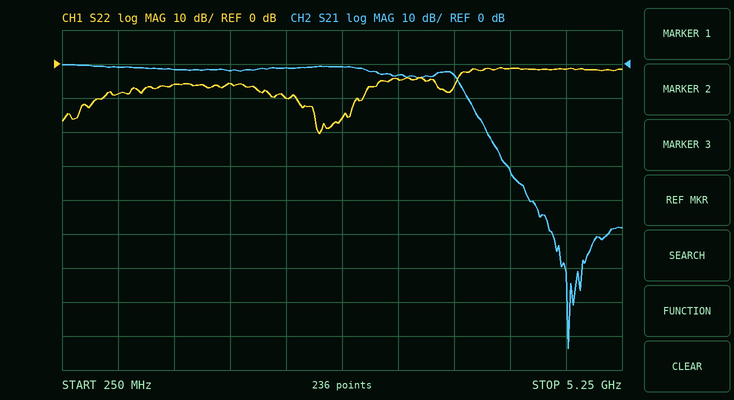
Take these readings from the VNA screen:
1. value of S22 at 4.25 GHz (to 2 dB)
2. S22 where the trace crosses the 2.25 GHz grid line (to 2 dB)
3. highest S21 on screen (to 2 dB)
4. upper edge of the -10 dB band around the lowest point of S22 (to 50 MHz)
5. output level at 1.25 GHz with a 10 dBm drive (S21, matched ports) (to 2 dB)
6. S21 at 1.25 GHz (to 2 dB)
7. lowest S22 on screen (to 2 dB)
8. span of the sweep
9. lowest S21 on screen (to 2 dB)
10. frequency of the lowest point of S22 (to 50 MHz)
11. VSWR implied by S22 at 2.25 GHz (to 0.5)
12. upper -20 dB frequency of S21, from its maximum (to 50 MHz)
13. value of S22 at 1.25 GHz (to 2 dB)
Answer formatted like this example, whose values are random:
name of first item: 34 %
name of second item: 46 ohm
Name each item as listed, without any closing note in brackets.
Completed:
value of S22 at 4.25 GHz: -2 dB
S22 where the trace crosses the 2.25 GHz grid line: -10 dB
highest S21 on screen: 0 dB
upper edge of the -10 dB band around the lowest point of S22: 2.95 GHz
output level at 1.25 GHz with a 10 dBm drive (S21, matched ports): 8 dBm
S21 at 1.25 GHz: -2 dB
lowest S22 on screen: -20 dB
span of the sweep: 5 GHz
lowest S21 on screen: -84 dB
frequency of the lowest point of S22: 2.55 GHz
VSWR implied by S22 at 2.25 GHz: 2.0
upper -20 dB frequency of S21, from its maximum: 4.05 GHz
value of S22 at 1.25 GHz: -6 dB
